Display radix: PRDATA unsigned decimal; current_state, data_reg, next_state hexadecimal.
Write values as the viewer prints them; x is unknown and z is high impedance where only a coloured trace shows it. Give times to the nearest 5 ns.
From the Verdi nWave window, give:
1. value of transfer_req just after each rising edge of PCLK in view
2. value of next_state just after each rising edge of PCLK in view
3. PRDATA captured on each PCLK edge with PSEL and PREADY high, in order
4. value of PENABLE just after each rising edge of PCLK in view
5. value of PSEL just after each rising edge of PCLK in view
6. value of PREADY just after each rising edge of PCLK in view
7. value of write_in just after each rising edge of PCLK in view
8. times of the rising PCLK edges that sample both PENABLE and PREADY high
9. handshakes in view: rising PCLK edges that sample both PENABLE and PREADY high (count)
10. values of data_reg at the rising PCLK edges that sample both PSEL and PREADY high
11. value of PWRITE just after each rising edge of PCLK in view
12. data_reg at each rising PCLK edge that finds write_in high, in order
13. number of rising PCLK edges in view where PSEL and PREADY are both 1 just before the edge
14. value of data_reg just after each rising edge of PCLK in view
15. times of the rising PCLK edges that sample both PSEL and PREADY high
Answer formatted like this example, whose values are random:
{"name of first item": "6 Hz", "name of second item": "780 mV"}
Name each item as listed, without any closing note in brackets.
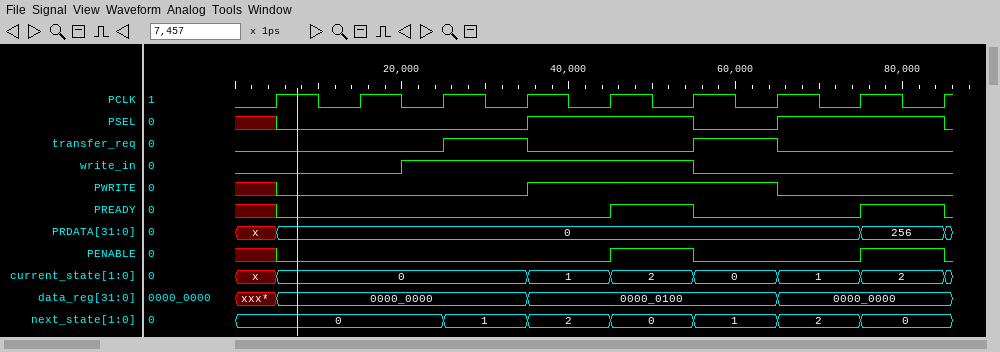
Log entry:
{"value of transfer_req just after each rising edge of PCLK in view": "0 0 1 0 0 1 0 0 0", "value of next_state just after each rising edge of PCLK in view": "0, 0, 1, 2, 0, 1, 2, 0, 0", "PRDATA captured on each PCLK edge with PSEL and PREADY high, in order": "0, 256", "value of PENABLE just after each rising edge of PCLK in view": "0 0 0 0 1 0 0 1 0", "value of PSEL just after each rising edge of PCLK in view": "0 0 0 1 1 0 1 1 0", "value of PREADY just after each rising edge of PCLK in view": "0 0 0 0 1 0 0 1 0", "value of write_in just after each rising edge of PCLK in view": "0 0 1 1 1 0 0 0 0", "times of the rising PCLK edges that sample both PENABLE and PREADY high": "55 ns, 85 ns", "handshakes in view: rising PCLK edges that sample both PENABLE and PREADY high": "2", "values of data_reg at the rising PCLK edges that sample both PSEL and PREADY high": "0000_0100, 0000_0000", "value of PWRITE just after each rising edge of PCLK in view": "0 0 0 1 1 1 0 0 0", "data_reg at each rising PCLK edge that finds write_in high, in order": "0000_0000, 0000_0000, 0000_0100, 0000_0100", "number of rising PCLK edges in view where PSEL and PREADY are both 1 just before the edge": "2", "value of data_reg just after each rising edge of PCLK in view": "0000_0000, 0000_0000, 0000_0000, 0000_0100, 0000_0100, 0000_0100, 0000_0000, 0000_0000, 0000_0000", "times of the rising PCLK edges that sample both PSEL and PREADY high": "55 ns, 85 ns"}
